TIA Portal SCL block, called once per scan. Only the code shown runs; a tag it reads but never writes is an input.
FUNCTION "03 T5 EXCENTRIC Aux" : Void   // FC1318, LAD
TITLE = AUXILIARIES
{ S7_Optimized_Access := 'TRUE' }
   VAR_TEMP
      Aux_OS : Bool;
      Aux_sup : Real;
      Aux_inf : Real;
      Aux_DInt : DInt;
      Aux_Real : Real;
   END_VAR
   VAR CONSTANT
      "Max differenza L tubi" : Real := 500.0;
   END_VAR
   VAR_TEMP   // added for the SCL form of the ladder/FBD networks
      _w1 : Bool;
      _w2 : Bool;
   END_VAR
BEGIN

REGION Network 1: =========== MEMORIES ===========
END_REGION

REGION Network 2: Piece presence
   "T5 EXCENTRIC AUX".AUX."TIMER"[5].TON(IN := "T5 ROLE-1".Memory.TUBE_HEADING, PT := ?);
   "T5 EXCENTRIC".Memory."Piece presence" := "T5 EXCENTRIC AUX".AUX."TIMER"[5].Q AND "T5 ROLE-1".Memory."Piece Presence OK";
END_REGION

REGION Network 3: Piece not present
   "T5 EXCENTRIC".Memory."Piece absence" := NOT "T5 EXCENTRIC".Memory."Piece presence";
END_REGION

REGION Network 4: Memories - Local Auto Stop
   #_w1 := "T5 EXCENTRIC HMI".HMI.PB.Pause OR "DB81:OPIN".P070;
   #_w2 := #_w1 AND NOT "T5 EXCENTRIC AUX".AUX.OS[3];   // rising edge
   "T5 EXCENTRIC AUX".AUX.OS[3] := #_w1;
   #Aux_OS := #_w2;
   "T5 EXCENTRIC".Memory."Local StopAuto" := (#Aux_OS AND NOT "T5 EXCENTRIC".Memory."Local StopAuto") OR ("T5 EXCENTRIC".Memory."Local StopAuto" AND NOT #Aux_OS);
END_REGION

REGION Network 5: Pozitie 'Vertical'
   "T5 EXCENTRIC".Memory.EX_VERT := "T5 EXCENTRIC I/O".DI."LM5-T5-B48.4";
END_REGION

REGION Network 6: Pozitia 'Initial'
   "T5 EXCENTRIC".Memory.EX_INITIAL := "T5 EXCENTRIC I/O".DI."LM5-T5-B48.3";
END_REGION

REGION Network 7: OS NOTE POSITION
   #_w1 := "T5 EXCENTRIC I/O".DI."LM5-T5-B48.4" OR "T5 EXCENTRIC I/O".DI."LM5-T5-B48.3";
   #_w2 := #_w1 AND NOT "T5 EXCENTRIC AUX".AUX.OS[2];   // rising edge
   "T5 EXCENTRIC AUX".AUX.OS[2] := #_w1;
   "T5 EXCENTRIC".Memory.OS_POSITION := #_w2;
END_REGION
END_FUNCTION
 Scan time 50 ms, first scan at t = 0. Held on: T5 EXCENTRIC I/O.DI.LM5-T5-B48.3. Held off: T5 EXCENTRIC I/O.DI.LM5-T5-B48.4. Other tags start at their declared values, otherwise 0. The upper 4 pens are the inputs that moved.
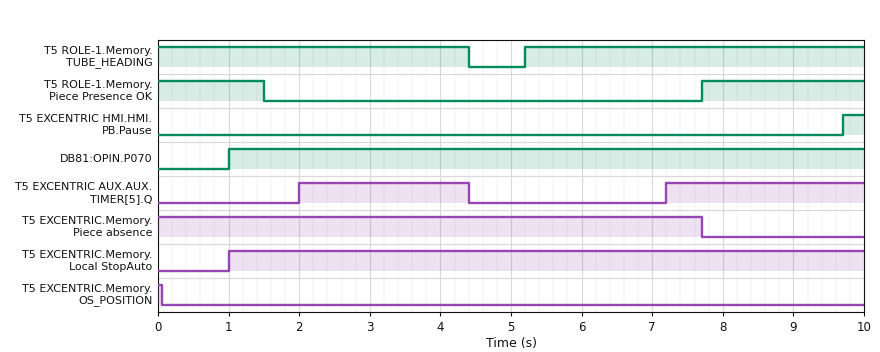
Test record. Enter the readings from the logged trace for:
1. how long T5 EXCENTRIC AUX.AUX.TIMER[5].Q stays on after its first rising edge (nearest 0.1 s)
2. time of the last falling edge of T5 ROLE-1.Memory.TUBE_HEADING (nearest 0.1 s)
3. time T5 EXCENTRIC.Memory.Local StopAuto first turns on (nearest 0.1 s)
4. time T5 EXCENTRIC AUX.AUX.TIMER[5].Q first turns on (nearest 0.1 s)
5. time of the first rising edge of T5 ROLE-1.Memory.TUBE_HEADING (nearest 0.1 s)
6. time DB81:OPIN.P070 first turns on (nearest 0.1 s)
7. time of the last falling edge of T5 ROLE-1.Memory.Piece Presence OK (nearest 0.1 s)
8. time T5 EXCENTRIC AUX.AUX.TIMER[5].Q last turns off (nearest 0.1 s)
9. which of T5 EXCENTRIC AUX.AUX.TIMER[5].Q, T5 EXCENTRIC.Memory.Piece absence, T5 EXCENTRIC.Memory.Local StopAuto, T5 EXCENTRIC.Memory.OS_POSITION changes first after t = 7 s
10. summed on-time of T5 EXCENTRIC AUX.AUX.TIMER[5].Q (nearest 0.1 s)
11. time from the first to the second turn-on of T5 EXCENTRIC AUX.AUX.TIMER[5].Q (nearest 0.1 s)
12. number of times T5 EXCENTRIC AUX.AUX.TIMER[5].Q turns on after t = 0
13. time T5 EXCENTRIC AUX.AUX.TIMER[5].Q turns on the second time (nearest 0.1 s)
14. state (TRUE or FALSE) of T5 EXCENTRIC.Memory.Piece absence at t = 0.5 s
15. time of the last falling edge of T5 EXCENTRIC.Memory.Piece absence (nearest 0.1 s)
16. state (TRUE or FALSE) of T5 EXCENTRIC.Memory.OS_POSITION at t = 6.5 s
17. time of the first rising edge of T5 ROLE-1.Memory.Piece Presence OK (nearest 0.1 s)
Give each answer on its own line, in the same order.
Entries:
2.4 s
4.4 s
1.0 s
2.0 s
5.2 s
1.0 s
1.5 s
4.4 s
T5 EXCENTRIC AUX.AUX.TIMER[5].Q
5.2 s
5.2 s
2
7.2 s
TRUE
7.7 s
FALSE
7.7 s
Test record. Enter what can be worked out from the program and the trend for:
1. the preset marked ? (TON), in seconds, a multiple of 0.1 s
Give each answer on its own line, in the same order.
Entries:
2.0 s
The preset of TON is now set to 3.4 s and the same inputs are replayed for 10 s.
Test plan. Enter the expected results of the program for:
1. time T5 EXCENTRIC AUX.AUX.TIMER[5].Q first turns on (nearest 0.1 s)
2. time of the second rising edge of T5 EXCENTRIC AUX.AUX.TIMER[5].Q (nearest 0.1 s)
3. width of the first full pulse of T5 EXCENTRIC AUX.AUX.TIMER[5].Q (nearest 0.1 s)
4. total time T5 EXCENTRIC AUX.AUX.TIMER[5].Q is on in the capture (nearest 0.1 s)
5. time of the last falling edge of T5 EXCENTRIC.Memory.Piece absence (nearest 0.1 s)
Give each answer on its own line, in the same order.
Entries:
3.4 s
8.6 s
1.0 s
2.4 s
8.6 s
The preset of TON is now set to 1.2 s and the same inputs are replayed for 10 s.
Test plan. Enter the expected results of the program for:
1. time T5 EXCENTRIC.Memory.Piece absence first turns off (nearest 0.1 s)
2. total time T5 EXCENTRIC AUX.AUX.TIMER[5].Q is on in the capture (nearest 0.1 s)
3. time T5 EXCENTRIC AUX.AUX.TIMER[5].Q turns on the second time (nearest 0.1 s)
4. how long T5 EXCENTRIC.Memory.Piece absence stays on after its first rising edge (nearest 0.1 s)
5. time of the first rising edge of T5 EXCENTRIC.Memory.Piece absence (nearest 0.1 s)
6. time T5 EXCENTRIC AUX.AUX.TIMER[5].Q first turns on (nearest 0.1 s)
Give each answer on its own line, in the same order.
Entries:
1.2 s
6.8 s
6.4 s
6.2 s
1.5 s
1.2 s
